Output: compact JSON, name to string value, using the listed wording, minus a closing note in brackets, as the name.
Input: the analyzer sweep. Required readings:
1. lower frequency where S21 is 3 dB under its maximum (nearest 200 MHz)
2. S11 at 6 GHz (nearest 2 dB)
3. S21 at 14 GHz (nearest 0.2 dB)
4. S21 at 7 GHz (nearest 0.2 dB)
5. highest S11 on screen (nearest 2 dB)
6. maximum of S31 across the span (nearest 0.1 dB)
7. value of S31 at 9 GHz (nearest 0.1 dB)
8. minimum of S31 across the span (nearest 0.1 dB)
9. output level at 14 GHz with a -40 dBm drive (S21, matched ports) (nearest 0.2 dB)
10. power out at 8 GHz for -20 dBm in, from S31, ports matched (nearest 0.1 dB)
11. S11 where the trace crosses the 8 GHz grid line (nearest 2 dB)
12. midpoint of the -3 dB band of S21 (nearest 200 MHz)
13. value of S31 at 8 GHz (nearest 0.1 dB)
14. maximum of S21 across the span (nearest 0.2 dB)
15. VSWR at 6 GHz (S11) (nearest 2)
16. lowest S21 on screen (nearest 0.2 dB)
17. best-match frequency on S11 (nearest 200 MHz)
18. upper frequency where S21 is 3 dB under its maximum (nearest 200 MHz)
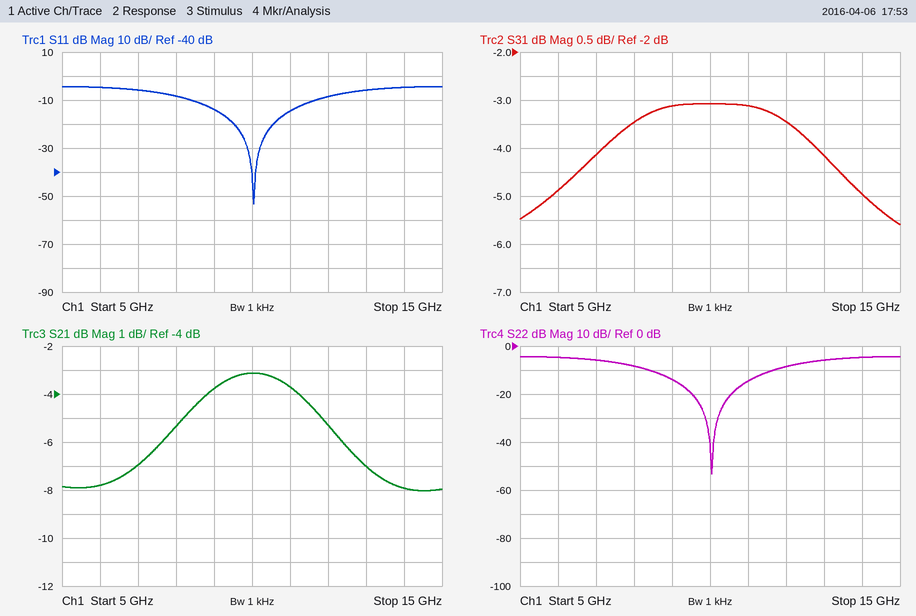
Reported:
{"lower frequency where S21 is 3 dB under its maximum": "7.6 GHz", "S11 at 6 GHz": "-4 dB", "S21 at 14 GHz": "-8.0 dB", "S21 at 7 GHz": "-7.0 dB", "highest S11 on screen": "-4 dB", "maximum of S31 across the span": "-3.1 dB", "value of S31 at 9 GHz": "-3.1 dB", "minimum of S31 across the span": "-5.6 dB", "output level at 14 GHz with a -40 dBm drive (S21, matched ports)": "-48.0 dBm", "power out at 8 GHz for -20 dBm in, from S31, ports matched": "-23.5 dBm", "S11 where the trace crosses the 8 GHz grid line": "-8 dB", "midpoint of the -3 dB band of S21": "10.0 GHz", "value of S31 at 8 GHz": "-3.5 dB", "maximum of S21 across the span": "-3.2 dB", "VSWR at 6 GHz (S11)": "4", "lowest S21 on screen": "-8.0 dB", "best-match frequency on S11": "10.0 GHz", "upper frequency where S21 is 3 dB under its maximum": "12.4 GHz"}
